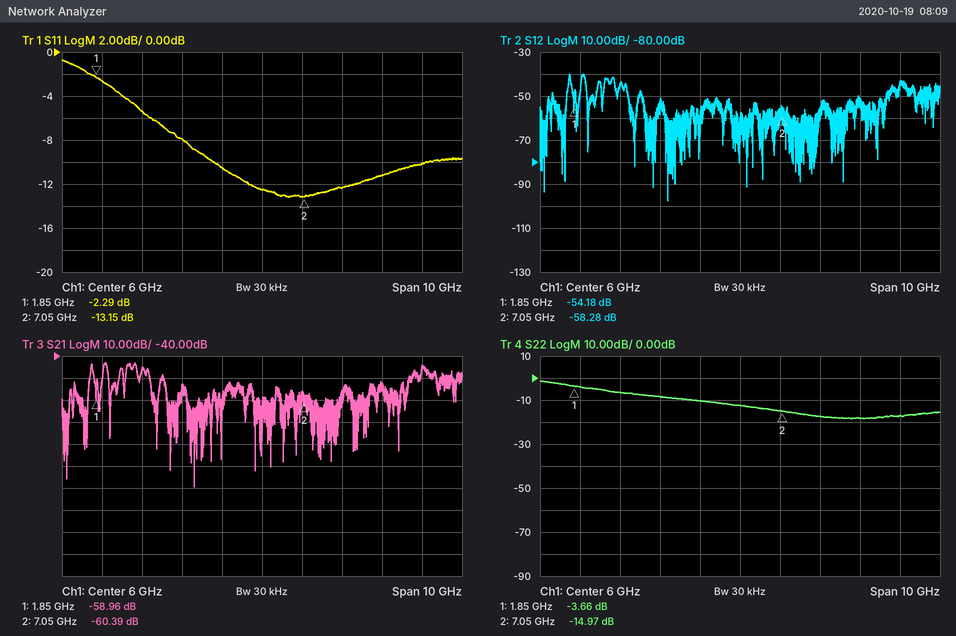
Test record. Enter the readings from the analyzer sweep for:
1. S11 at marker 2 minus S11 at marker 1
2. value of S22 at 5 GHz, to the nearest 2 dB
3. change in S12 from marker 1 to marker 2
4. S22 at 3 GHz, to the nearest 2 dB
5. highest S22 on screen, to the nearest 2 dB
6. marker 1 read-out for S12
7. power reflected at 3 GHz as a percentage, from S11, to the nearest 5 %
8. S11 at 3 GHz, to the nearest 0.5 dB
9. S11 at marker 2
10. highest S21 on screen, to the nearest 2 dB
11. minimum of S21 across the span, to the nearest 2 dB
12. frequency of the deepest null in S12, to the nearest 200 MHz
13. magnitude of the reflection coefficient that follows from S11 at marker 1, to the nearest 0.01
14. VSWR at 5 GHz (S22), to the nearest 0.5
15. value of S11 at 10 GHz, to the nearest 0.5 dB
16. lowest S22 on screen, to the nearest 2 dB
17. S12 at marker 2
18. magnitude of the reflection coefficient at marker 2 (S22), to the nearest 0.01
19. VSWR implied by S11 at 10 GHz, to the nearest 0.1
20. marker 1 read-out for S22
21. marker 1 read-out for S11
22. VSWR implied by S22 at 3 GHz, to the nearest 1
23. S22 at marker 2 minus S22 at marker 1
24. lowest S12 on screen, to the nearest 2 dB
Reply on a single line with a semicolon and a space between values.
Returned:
-10.86 dB; -10 dB; -4.10 dB; -6 dB; -2 dB; -54.18 dB; 30 %; -5.5 dB; -13.15 dB; -42 dB; -100 dB; 4.2 GHz; 0.77; 2.0; -10.0 dB; -18 dB; -58.28 dB; 0.18; 1.9; -3.66 dB; -2.29 dB; 3; -11.31 dB; -98 dB
